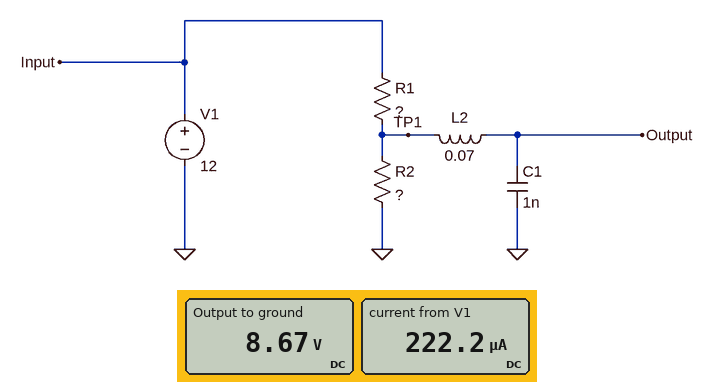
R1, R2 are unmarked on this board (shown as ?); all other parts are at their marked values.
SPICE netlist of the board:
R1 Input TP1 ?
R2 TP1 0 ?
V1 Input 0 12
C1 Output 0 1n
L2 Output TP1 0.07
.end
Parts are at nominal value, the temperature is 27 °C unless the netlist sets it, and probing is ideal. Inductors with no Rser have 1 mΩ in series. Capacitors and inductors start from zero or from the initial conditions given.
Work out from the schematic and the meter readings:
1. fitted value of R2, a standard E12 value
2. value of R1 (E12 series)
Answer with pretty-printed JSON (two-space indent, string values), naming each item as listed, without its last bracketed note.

{
  "fitted value of R2, a standard E12 value": "39 kΩ",
  "value of R1": "15 kΩ"
}
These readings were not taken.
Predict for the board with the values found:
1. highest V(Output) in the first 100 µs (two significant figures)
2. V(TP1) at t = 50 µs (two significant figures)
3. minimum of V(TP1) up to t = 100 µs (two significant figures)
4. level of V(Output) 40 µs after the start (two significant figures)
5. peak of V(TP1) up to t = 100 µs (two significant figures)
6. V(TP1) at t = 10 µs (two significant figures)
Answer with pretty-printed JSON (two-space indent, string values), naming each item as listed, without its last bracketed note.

{
  "highest V(Output) in the first 100 µs": "9.3 V",
  "V(TP1) at t = 50 µs": "9.0 V",
  "minimum of V(TP1) up to t = 100 µs": "3.3 V",
  "level of V(Output) 40 µs after the start": "9.2 V",
  "peak of V(TP1) up to t = 100 µs": "9.0 V",
  "V(TP1) at t = 10 µs": "3.3 V"
}
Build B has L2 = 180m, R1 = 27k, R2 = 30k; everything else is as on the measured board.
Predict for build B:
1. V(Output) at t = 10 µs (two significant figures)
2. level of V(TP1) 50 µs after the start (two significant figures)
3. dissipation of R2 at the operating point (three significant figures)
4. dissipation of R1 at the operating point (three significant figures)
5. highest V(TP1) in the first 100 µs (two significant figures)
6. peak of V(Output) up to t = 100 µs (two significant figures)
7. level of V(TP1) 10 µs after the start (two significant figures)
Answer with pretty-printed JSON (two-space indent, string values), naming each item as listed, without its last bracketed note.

{
  "V(Output) at t = 10 µs": "1.3 V",
  "level of V(TP1) 50 µs after the start": "6.3 V",
  "dissipation of R2 at the operating point": "1.33 mW",
  "dissipation of R1 at the operating point": "1.20 mW",
  "highest V(TP1) in the first 100 µs": "6.8 V",
  "peak of V(Output) up to t = 100 µs": "7.2 V",
  "level of V(TP1) 10 µs after the start": "3.2 V"
}
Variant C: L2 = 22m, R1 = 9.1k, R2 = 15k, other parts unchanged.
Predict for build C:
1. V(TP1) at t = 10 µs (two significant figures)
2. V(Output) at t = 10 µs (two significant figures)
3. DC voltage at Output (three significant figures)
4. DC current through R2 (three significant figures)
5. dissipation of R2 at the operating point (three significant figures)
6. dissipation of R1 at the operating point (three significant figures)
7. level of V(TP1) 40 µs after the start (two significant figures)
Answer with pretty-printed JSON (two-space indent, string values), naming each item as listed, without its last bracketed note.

{
  "V(TP1) at t = 10 µs": "4.4 V",
  "V(Output) at t = 10 µs": "6.2 V",
  "DC voltage at Output": "7.47 V",
  "DC current through R2": "498 µA",
  "dissipation of R2 at the operating point": "3.72 mW",
  "dissipation of R1 at the operating point": "2.26 mW",
  "level of V(TP1) 40 µs after the start": "7.4 V"
}
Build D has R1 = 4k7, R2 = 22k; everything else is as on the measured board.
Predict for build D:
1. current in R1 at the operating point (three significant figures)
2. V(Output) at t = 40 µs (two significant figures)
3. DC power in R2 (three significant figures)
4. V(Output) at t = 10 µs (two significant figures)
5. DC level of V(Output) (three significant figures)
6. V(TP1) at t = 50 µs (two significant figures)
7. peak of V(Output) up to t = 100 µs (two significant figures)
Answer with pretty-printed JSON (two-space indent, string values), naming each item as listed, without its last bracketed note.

{
  "current in R1 at the operating point": "449 µA",
  "V(Output) at t = 40 µs": "11 V",
  "DC power in R2": "4.44 mW",
  "V(Output) at t = 10 µs": "5.3 V",
  "DC level of V(Output)": "9.89 V",
  "V(TP1) at t = 50 µs": "10 V",
  "peak of V(Output) up to t = 100 µs": "15 V"
}
